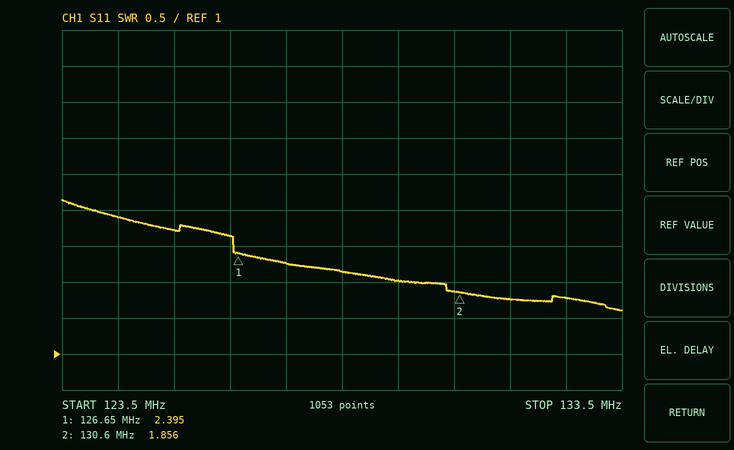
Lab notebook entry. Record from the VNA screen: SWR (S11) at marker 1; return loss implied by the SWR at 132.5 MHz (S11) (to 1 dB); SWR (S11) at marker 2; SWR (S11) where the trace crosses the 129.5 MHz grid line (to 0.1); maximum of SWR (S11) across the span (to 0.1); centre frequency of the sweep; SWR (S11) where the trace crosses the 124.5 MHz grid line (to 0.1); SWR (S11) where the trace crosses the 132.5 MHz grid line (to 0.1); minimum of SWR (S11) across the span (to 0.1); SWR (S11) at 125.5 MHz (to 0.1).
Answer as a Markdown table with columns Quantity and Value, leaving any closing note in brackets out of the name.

| Quantity | Value |
|---|---|
| SWR (S11) at marker 1 | 2.395 |
| return loss implied by the SWR at 132.5 MHz (S11) | 11 dB |
| SWR (S11) at marker 2 | 1.856 |
| SWR (S11) where the trace crosses the 129.5 MHz grid line | 2.0 |
| maximum of SWR (S11) across the span | 3.1 |
| centre frequency of the sweep | 128.5 MHz |
| SWR (S11) where the trace crosses the 124.5 MHz grid line | 2.9 |
| SWR (S11) where the trace crosses the 132.5 MHz grid line | 1.8 |
| minimum of SWR (S11) across the span | 1.6 |
| SWR (S11) at 125.5 MHz | 2.7 |
